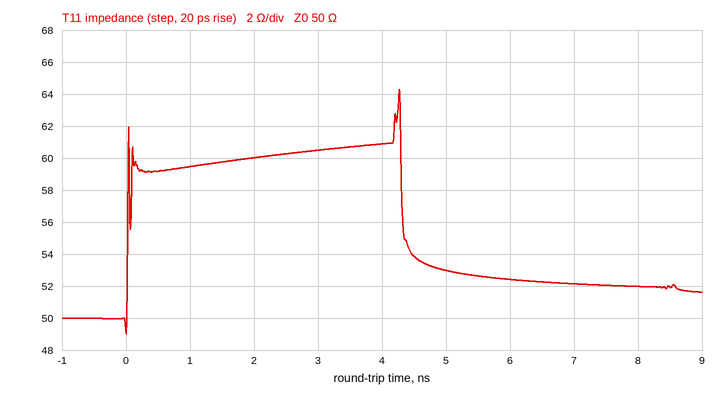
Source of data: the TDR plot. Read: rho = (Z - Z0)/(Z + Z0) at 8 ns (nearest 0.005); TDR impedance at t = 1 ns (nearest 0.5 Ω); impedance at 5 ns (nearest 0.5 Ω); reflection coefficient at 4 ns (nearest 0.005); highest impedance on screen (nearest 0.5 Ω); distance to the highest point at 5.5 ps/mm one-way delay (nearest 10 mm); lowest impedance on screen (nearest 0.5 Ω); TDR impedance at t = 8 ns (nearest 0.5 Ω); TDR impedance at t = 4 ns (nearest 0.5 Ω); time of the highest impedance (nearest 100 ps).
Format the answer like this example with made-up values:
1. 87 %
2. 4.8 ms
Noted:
1. +0.020
2. 59.5 Ω
3. 53.0 Ω
4. +0.100
5. 64.5 Ω
6. 390 mm
7. 49.0 Ω
8. 52.0 Ω
9. 61.0 Ω
10. 4.3 ns
